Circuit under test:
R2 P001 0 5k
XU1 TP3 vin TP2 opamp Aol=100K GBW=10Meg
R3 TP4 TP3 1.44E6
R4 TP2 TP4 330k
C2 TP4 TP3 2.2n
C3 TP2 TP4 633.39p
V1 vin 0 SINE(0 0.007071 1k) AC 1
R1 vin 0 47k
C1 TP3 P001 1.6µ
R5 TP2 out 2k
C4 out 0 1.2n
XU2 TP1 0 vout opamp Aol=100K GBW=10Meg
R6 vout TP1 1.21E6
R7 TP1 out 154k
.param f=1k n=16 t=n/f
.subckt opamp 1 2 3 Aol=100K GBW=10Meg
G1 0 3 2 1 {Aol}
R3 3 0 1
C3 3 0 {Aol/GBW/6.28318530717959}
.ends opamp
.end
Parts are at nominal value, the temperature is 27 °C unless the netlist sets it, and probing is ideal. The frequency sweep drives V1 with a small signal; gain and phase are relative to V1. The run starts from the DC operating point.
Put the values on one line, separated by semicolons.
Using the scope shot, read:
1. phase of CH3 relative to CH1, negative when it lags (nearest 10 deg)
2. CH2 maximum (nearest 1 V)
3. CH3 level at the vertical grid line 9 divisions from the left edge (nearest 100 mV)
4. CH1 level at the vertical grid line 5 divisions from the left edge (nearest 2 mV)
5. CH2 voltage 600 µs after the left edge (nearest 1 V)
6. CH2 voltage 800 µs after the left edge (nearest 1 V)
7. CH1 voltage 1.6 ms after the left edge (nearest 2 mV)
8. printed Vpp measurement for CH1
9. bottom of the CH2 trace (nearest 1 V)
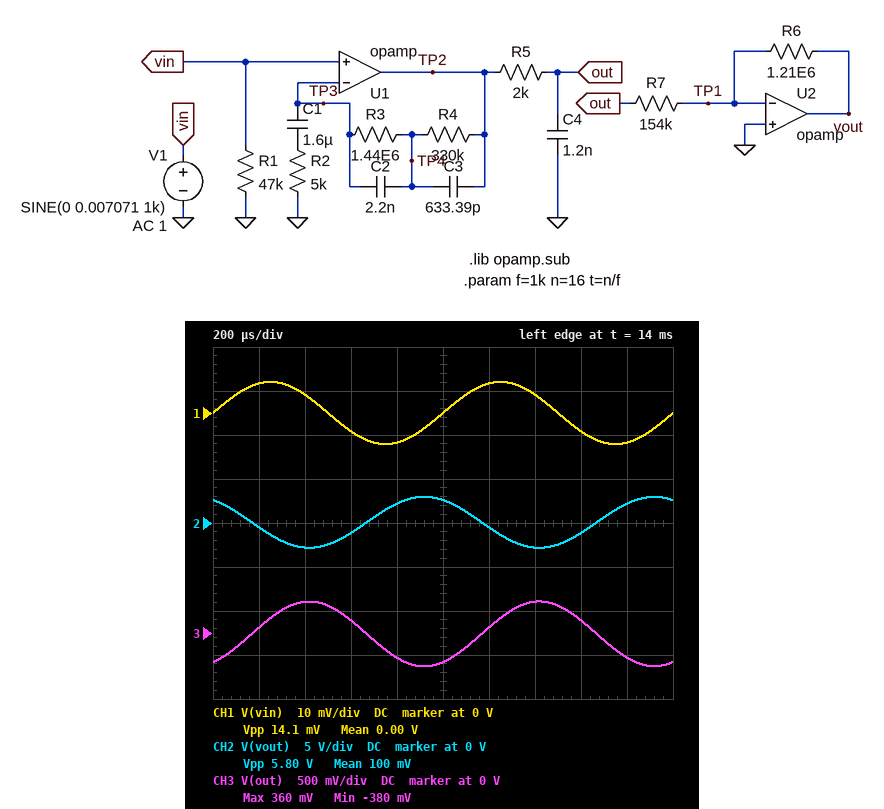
-60 deg; 3 V; -300 mV; 0 V; -1 V; 2 V; -4 mV; 14.1 mV; -3 V
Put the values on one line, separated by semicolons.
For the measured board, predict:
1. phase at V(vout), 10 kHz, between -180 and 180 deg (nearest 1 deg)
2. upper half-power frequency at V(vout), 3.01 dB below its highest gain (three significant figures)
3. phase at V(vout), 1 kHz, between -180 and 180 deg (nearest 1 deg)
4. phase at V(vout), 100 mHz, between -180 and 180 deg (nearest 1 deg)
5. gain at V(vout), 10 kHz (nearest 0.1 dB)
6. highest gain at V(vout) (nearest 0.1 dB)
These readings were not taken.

93 deg; 90.9 Hz; 119 deg; -120 deg; 34.0 dB; 66.0 dB
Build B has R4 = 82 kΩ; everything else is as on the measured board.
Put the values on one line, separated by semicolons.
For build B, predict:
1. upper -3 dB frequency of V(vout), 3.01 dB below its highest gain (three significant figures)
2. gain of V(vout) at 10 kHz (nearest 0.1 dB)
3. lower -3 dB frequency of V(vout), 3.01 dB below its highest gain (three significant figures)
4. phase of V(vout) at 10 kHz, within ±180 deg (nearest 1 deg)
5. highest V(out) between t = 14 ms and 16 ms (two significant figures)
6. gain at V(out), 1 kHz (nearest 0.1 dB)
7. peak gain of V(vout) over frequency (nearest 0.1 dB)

83.0 Hz; 33.9 dB; 12.1 Hz; 103 deg; 170 mV; 28.0 dB; 64.6 dB
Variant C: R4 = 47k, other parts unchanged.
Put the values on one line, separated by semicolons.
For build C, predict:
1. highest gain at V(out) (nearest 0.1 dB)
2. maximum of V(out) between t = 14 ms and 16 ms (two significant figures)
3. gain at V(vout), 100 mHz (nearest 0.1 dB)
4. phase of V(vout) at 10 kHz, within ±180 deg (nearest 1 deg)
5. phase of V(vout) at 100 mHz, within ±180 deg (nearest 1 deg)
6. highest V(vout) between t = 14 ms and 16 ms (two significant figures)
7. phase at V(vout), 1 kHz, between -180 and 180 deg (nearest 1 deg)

46.5 dB; 130 mV; 22.9 dB; 111 deg; -124 deg; 1.1 V; 124 deg
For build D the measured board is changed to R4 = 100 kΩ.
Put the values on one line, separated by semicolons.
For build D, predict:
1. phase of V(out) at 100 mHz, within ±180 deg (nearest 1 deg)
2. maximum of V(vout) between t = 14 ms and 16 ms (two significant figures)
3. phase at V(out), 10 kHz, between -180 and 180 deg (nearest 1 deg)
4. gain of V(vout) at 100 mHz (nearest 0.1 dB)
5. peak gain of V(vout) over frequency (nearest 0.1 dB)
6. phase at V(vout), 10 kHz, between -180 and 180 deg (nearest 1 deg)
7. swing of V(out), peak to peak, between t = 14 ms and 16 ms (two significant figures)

57 deg; 1.6 V; -79 deg; 23.1 dB; 64.7 dB; 101 deg; 400 mV
